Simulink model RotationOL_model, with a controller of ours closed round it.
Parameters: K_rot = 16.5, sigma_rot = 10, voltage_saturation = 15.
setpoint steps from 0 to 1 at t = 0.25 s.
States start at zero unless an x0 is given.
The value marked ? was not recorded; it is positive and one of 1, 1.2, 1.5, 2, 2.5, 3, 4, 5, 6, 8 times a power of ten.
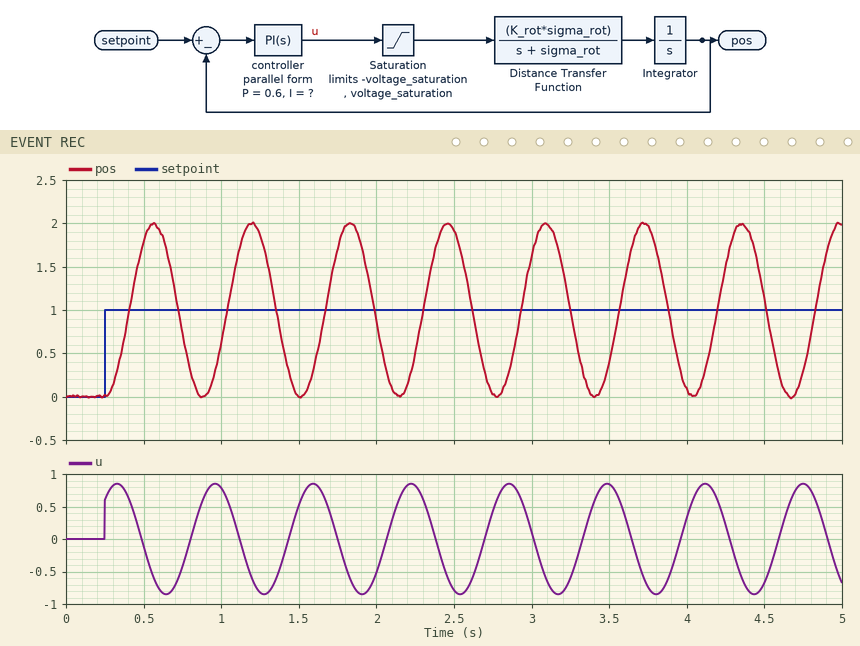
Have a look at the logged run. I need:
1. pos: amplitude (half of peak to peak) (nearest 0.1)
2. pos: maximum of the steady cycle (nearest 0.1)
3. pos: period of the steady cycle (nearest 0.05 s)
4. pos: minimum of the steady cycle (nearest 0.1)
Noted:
1.0
2.0
0.65 s
0.0
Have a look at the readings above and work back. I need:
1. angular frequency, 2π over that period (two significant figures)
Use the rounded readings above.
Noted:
9.7 rad/s
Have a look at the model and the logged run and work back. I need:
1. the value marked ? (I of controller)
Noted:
6
